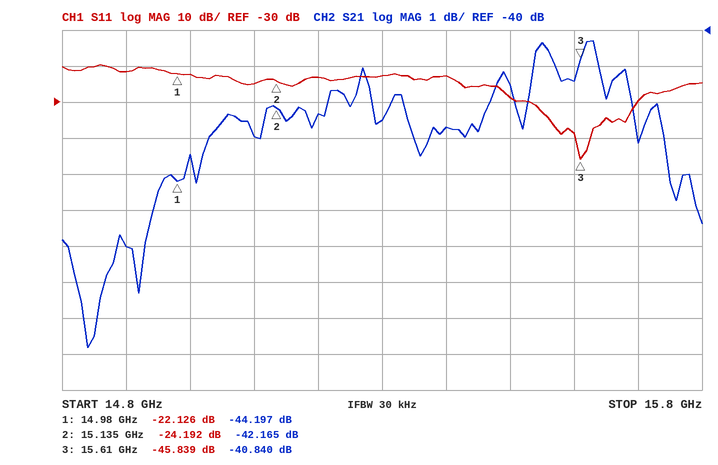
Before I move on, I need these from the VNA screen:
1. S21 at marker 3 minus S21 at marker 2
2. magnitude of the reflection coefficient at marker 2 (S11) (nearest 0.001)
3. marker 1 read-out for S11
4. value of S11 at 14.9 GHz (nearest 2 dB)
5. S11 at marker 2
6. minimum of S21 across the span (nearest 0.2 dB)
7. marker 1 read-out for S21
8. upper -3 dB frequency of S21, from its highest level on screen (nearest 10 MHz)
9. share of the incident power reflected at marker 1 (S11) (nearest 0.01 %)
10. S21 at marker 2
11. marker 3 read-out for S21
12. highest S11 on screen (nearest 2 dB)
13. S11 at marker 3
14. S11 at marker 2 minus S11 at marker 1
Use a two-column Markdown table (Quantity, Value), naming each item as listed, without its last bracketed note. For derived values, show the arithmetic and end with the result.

| Quantity | Value |
|---|---|
| S21 at marker 3 minus S21 at marker 2 | -40.84 − (-42.165) = 1.325 dB |
| magnitude of the reflection coefficient at marker 2 (S11) | 10^(-24.192/20) ≈ 0.062 |
| marker 1 read-out for S11 | -22.126 dB |
| value of S11 at 14.9 GHz | -22 dB |
| S11 at marker 2 | -24.192 dB |
| minimum of S21 across the span | -48.8 dB |
| marker 1 read-out for S21 | -44.197 dB |
| upper -3 dB frequency of S21, from its highest level on screen | 15.74 GHz |
| share of the incident power reflected at marker 1 (S11) | 10^(-22.126/10) ≈ 0.61 % |
| S21 at marker 2 | -42.165 dB |
| marker 3 read-out for S21 | -40.840 dB |
| highest S11 on screen | -20 dB |
| S11 at marker 3 | -45.839 dB |
| S11 at marker 2 minus S11 at marker 1 | -24.192 − (-22.126) = -2.066 dB |
